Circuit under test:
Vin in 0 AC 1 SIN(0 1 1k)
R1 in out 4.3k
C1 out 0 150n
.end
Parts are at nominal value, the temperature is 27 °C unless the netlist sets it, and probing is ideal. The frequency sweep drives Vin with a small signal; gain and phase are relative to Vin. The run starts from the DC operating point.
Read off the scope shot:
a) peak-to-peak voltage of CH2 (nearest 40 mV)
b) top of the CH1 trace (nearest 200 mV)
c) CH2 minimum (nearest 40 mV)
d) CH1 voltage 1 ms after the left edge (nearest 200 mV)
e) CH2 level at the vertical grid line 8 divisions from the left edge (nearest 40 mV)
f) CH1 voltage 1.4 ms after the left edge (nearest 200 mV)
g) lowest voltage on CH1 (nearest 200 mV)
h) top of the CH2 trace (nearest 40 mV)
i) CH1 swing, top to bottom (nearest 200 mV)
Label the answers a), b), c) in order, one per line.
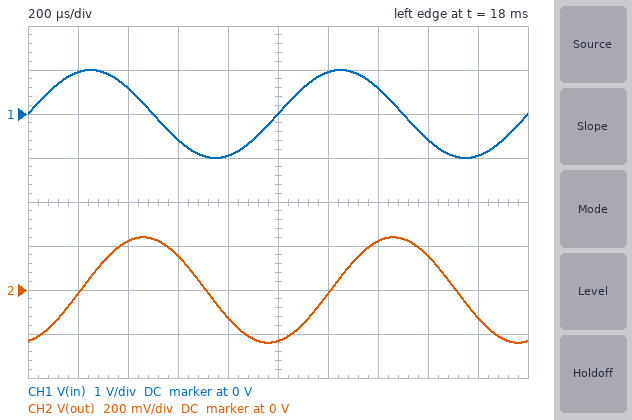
a) 480 mV
b) 1.0 V
c) -240 mV
d) 0 V
e) 160 mV
f) 600 mV
g) -1.0 V
h) 240 mV
i) 2.0 V
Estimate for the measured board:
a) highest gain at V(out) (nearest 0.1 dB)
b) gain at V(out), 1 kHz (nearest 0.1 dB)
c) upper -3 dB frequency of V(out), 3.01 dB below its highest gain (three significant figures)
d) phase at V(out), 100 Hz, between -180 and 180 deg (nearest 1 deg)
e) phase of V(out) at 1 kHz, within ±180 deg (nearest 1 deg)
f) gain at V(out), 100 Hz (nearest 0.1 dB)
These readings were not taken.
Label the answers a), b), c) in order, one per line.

a) 0 dB
b) -12.4 dB
c) 247 Hz
d) -22 deg
e) -76 deg
f) -0.7 dB
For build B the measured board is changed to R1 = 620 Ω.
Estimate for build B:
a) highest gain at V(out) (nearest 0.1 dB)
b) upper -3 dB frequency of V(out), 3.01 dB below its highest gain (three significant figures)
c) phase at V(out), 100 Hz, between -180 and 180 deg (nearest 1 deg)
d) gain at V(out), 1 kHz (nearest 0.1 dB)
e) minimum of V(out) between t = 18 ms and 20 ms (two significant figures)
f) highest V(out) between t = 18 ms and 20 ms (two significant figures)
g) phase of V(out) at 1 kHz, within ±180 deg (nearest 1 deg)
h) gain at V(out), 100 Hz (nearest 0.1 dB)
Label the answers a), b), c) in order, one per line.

a) 0 dB
b) 1.71 kHz
c) -3 deg
d) -1.3 dB
e) -860 mV
f) 860 mV
g) -30 deg
h) 0 dB
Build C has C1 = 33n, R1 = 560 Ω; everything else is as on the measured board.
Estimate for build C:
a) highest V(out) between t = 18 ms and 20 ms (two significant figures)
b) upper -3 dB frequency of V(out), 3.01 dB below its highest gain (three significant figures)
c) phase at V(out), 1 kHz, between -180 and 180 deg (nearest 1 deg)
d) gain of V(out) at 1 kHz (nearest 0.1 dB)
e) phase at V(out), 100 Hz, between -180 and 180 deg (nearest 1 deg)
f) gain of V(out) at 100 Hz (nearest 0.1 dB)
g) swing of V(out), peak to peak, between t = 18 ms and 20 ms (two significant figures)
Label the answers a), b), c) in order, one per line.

a) 990 mV
b) 8.61 kHz
c) -7 deg
d) -0.1 dB
e) -1 deg
f) 0 dB
g) 2.0 V
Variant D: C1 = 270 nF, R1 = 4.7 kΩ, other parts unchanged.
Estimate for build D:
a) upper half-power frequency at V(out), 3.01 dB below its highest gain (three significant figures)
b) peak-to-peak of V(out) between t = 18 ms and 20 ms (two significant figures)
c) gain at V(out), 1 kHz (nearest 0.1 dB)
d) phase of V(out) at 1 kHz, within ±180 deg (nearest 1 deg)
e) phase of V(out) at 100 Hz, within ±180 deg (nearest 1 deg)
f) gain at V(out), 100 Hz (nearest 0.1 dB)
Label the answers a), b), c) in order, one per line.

a) 125 Hz
b) 250 mV
c) -18.1 dB
d) -83 deg
e) -39 deg
f) -2.1 dB
